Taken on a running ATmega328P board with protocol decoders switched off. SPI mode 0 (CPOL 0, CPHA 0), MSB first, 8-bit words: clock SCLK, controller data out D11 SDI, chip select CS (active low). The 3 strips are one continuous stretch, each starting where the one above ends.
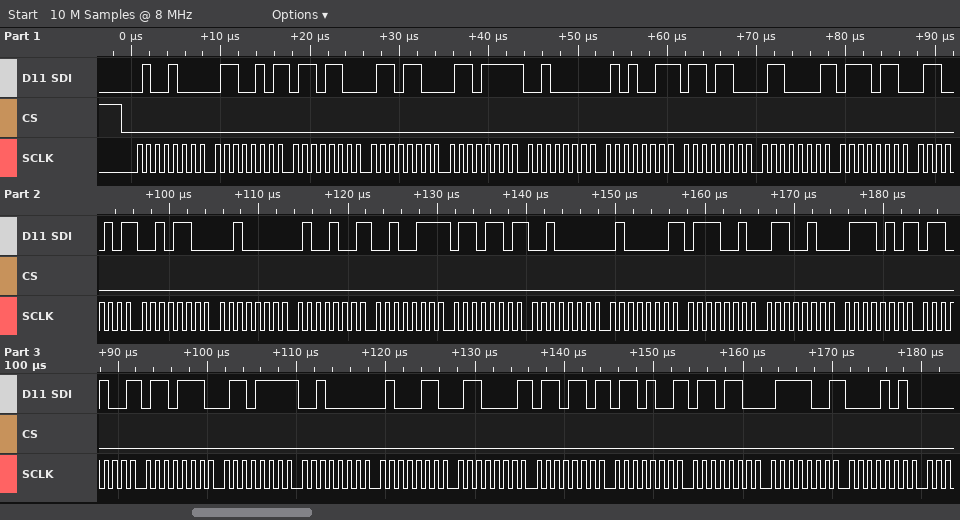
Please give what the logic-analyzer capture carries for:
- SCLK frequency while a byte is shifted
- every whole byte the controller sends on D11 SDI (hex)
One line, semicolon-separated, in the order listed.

1 MHz; 0x48 0x65 0x6C 0x6C 0x6F 0x20 0x53 0x6C 0x61 0x76 0x65 0x2C 0x20 0x49 0x27 0x6D 0x20 0x41 0x72 0x64 0x75 0x69 0x6E 0x6F 0x20 0x46 0x61 0x6D 0x69 0x6C 0x79 0x0A
